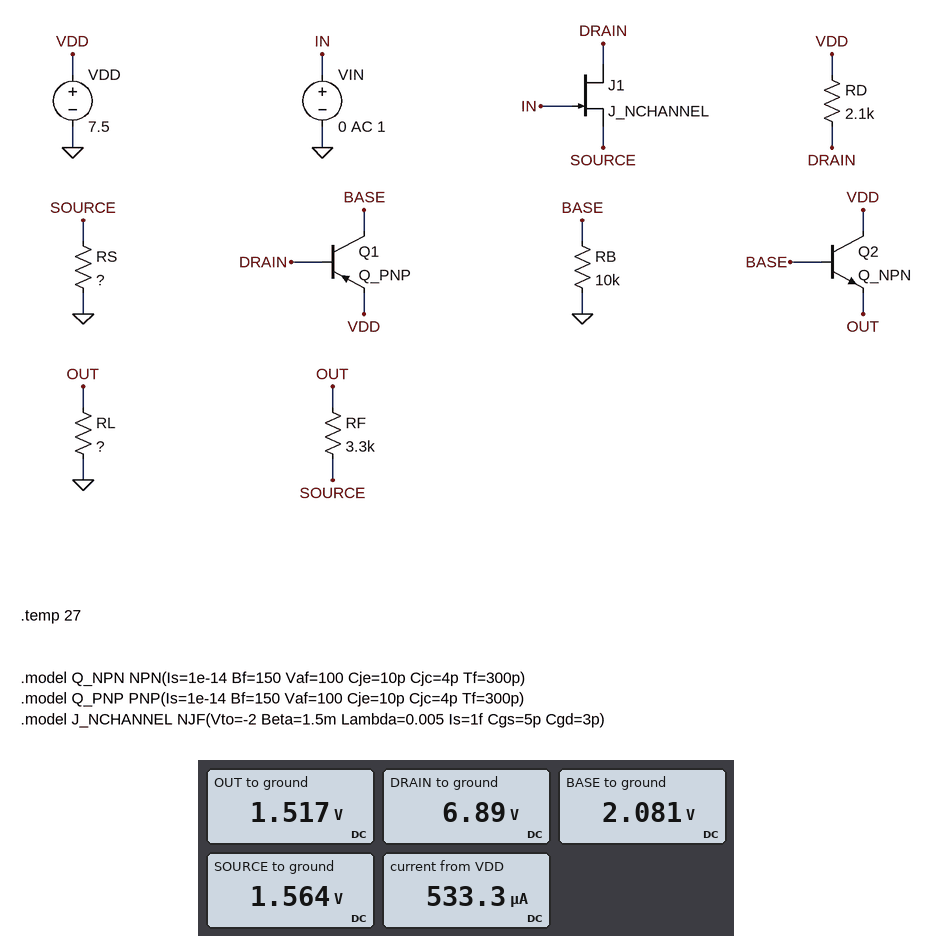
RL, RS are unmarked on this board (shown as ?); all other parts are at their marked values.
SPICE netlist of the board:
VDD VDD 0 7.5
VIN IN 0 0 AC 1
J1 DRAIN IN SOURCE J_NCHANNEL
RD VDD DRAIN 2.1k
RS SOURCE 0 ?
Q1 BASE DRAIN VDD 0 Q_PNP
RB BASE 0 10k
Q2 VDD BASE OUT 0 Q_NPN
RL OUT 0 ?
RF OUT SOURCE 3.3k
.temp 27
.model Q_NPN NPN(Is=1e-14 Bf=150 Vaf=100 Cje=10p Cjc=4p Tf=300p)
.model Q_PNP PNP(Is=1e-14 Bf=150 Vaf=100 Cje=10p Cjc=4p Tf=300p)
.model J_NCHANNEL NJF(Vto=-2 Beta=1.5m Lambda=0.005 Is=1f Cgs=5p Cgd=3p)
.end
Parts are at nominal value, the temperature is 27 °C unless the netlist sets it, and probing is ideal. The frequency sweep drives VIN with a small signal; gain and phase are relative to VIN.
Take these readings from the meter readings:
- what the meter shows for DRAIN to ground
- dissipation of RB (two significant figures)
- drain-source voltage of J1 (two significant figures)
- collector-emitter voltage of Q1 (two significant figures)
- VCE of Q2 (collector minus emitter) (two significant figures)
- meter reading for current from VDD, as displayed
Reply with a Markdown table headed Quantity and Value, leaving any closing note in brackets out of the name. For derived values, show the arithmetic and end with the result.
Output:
| Quantity | Value |
|---|---|
| what the meter shows for DRAIN to ground | 6.89 V |
| dissipation of RB | (2.081 V)^2 / 10 kΩ = 430 µW |
| drain-source voltage of J1 | 6.89 V - 1.564 V = 5.3 V |
| collector-emitter voltage of Q1 | 2.081 V - 7.5 V = -5.4 V |
| VCE of Q2 (collector minus emitter) | 7.5 V - 1.517 V = 6.0 V |
| meter reading for current from VDD, as displayed | 533.3 µA |
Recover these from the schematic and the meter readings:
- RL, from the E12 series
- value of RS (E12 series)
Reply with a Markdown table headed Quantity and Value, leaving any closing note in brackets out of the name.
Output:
| Quantity | Value |
|---|---|
| RL, from the E12 series | 33 kΩ |
| value of RS | 5.6 kΩ |
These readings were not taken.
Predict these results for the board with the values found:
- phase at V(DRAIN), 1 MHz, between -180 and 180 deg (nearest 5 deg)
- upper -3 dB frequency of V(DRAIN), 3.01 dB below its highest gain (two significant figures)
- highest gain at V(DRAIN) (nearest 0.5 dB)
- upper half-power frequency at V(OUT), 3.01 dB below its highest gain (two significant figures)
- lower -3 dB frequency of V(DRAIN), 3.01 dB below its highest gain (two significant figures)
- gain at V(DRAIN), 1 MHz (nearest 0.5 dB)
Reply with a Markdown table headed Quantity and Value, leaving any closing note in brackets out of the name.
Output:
| Quantity | Value |
|---|---|
| phase at V(DRAIN), 1 MHz, between -180 and 180 deg | -170 deg |
| upper -3 dB frequency of V(DRAIN), 3.01 dB below its highest gain | 220 MHz |
| highest gain at V(DRAIN) | -21.5 dB |
| upper half-power frequency at V(OUT), 3.01 dB below its highest gain | 16 MHz |
| lower -3 dB frequency of V(DRAIN), 3.01 dB below its highest gain | 7.8 MHz |
| gain at V(DRAIN), 1 MHz | -32.5 dB |
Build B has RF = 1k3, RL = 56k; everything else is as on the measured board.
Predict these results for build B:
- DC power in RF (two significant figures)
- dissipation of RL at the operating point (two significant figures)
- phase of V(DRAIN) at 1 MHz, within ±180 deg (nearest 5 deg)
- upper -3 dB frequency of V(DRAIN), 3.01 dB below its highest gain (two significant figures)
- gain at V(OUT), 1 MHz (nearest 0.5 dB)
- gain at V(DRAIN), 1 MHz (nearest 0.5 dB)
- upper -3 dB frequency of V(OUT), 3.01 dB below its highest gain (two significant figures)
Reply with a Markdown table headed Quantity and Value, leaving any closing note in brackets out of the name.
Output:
| Quantity | Value |
|---|---|
| DC power in RF | 260 nW |
| dissipation of RL at the operating point | 43 µW |
| phase of V(DRAIN) at 1 MHz, within ±180 deg | -165 deg |
| upper -3 dB frequency of V(DRAIN), 3.01 dB below its highest gain | 210 MHz |
| gain at V(OUT), 1 MHz | 1.5 dB |
| gain at V(DRAIN), 1 MHz | -33.0 dB |
| upper -3 dB frequency of V(OUT), 3.01 dB below its highest gain | 25 MHz |
